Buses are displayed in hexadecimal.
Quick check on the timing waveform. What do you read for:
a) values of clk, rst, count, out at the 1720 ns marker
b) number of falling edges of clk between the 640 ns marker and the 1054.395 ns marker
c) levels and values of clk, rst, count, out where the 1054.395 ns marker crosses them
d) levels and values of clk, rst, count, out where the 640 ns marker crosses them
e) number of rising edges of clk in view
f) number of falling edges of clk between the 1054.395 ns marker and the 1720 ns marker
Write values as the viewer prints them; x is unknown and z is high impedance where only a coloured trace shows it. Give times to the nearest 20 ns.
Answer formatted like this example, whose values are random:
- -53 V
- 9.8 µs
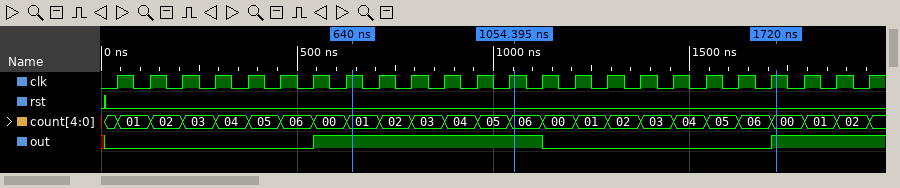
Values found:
- clk=1, rst=0, count=00, out=1
- 5
- clk=1, rst=0, count=06, out=1
- clk=1, rst=0, count=01, out=1
- 24
- 8
